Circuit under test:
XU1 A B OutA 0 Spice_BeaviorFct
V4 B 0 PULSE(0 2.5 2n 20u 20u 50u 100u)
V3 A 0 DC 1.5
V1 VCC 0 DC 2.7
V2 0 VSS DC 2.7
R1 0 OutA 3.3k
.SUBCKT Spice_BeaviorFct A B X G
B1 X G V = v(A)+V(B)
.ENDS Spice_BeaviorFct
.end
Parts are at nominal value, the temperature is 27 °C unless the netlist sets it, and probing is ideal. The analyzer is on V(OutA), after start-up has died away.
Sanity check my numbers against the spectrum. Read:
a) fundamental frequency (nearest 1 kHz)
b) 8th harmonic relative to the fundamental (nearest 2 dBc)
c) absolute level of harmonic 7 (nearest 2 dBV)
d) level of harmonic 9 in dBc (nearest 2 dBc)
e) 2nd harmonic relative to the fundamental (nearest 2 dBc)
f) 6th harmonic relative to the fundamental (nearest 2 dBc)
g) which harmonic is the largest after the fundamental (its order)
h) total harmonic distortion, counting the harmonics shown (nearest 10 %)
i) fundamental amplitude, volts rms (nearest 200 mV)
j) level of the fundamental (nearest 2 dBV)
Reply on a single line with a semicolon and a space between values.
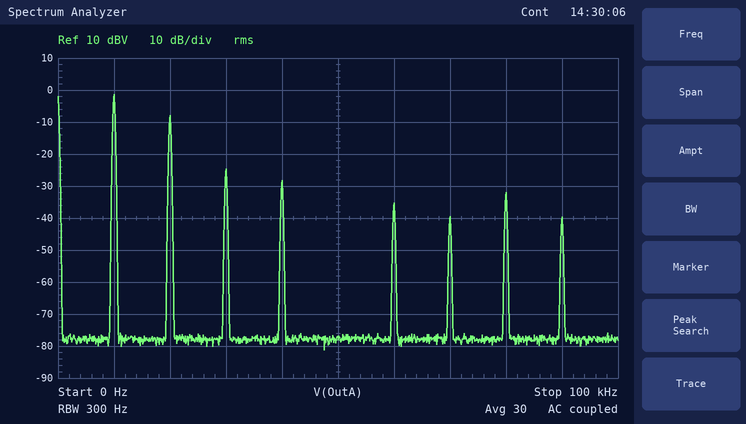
10 kHz; -30 dBc; -40 dBV; -38 dBc; -6 dBc; -34 dBc; 2; 50 %; 800 mV; -2 dBV
